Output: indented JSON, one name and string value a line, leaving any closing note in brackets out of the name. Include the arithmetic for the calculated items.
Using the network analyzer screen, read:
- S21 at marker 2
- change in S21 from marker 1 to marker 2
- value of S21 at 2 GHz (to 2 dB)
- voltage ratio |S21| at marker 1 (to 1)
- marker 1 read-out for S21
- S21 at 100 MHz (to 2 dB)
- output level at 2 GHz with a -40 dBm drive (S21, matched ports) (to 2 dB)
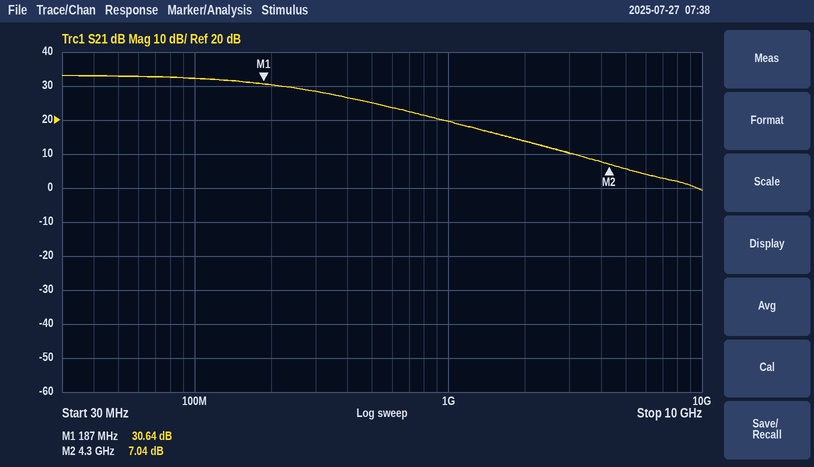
{
  "S21 at marker 2": "7.04 dB",
  "change in S21 from marker 1 to marker 2": "7.04 − (30.64) = -23.60 dB",
  "value of S21 at 2 GHz": "14 dB",
  "voltage ratio |S21| at marker 1": "10^(30.64/20) ≈ 34",
  "marker 1 read-out for S21": "30.64 dB",
  "S21 at 100 MHz": "32 dB",
  "output level at 2 GHz with a -40 dBm drive (S21, matched ports)": "-40 dBm + (14 dB) = -26 dBm"
}
